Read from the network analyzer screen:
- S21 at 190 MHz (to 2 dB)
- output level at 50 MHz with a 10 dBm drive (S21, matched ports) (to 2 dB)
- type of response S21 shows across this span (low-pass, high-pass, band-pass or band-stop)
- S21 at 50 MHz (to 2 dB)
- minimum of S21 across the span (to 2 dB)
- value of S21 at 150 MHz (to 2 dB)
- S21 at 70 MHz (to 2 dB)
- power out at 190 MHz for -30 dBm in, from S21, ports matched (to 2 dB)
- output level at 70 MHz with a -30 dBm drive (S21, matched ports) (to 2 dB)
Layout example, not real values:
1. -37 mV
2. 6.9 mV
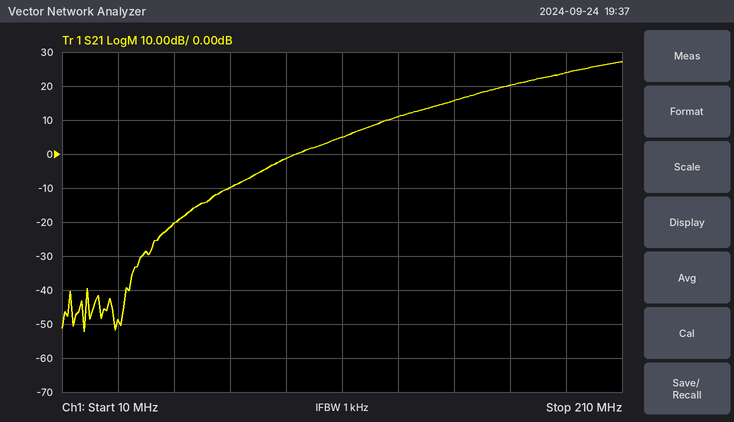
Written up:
1. 24 dB
2. -10 dBm
3. high-pass
4. -20 dB
5. -52 dB
6. 16 dB
7. -10 dB
8. -6 dBm
9. -40 dBm
